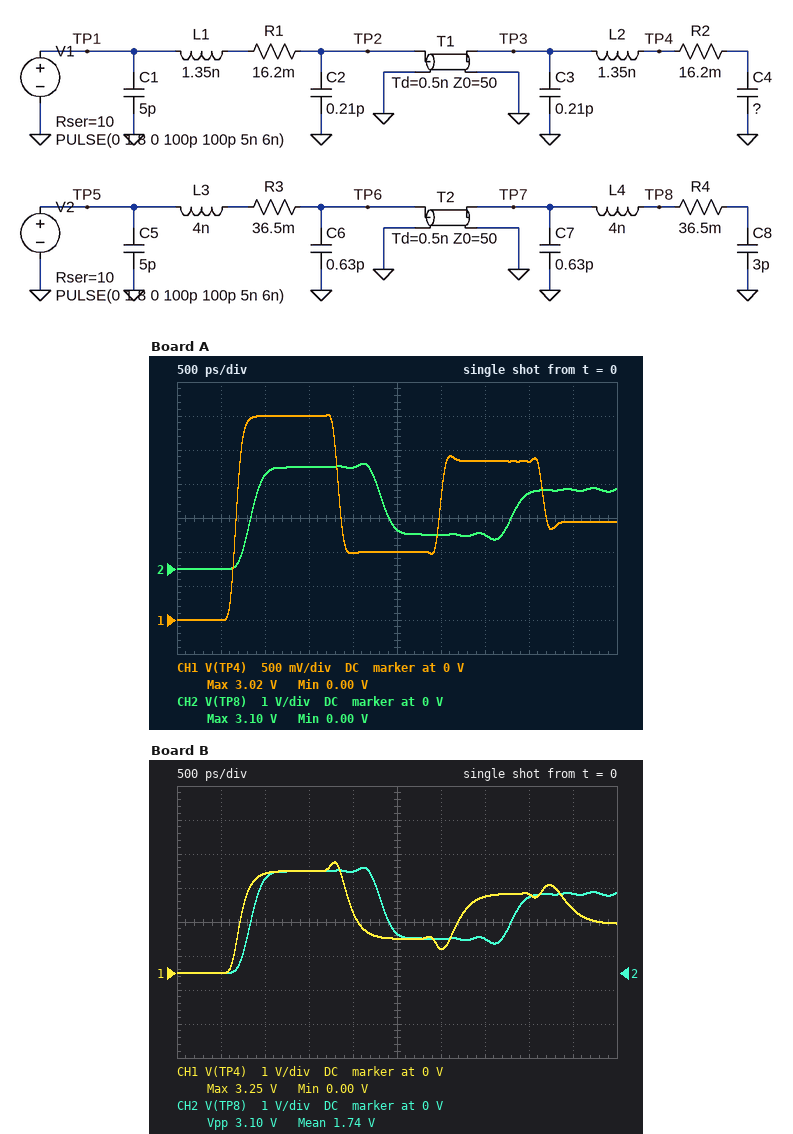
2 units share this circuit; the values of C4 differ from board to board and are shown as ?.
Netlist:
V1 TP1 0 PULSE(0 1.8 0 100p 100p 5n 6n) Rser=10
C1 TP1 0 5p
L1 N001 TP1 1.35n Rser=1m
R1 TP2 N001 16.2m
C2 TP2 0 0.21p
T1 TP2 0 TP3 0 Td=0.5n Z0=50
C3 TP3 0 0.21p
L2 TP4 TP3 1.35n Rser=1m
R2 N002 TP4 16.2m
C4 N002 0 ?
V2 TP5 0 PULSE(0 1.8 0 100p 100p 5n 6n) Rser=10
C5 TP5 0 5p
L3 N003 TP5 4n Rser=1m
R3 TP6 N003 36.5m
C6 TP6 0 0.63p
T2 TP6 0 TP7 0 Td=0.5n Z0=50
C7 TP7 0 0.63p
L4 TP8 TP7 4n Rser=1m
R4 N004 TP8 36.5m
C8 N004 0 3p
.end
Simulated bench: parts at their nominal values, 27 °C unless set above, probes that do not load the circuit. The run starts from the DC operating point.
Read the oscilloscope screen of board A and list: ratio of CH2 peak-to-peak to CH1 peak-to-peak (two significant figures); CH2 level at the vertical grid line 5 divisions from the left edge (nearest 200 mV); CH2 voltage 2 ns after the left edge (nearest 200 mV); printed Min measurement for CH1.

1.0
1.2 V
3.0 V
0.00 V
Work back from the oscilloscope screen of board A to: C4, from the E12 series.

1 pF
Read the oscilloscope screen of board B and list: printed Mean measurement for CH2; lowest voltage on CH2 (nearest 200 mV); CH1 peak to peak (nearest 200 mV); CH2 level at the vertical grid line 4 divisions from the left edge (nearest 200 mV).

1.74 V
0 V
3.2 V
3.0 V
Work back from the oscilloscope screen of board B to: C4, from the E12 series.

2.2 pF
